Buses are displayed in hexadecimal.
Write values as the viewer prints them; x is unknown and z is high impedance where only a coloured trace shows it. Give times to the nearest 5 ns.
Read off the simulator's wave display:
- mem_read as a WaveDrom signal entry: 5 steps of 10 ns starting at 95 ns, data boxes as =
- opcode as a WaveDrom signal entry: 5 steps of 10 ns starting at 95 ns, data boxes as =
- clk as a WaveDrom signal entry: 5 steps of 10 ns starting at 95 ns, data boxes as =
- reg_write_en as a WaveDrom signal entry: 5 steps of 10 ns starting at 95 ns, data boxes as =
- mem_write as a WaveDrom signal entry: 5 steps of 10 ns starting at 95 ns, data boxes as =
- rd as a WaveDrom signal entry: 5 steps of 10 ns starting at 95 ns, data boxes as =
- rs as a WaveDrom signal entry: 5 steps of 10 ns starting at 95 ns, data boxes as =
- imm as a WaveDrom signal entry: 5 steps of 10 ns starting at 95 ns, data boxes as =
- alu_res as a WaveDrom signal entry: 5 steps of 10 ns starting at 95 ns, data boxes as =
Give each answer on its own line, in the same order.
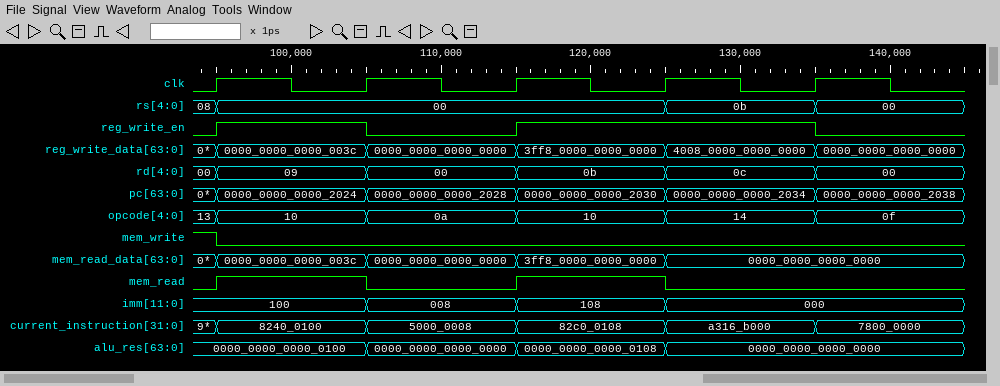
{name: 'mem_read', wave: '1010.'}
{name: 'opcode', wave: '=====', data: '10 0a 10 14 0f'}
{name: 'clk', wave: 'p....'}
{name: 'reg_write_en', wave: '101.0'}
{name: 'mem_write', wave: '0....'}
{name: 'rd', wave: '=====', data: '09 00 0b 0c 00'}
{name: 'rs', wave: '=..==', data: '00 0b 00'}
{name: 'imm', wave: '====.', data: '100 008 108 000'}
{name: 'alu_res', wave: '====.', data: '0000_0000_0000_0100 0000_0000_0000_0000 0000_0000_0000_0108 0000_0000_0000_0000'}
